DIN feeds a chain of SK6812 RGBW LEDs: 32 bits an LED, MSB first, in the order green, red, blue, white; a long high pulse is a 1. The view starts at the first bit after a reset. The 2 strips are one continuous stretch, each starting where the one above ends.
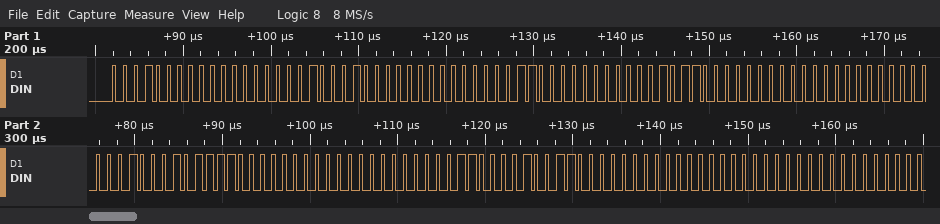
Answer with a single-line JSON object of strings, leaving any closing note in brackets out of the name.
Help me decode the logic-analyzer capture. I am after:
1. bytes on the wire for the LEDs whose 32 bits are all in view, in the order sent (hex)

{"bytes on the wire for the LEDs whose 32 bits are all in view, in the order sent": "10 00 22 00 06 00 2C 00 00 02 2F 00 00 0C 26 00"}
